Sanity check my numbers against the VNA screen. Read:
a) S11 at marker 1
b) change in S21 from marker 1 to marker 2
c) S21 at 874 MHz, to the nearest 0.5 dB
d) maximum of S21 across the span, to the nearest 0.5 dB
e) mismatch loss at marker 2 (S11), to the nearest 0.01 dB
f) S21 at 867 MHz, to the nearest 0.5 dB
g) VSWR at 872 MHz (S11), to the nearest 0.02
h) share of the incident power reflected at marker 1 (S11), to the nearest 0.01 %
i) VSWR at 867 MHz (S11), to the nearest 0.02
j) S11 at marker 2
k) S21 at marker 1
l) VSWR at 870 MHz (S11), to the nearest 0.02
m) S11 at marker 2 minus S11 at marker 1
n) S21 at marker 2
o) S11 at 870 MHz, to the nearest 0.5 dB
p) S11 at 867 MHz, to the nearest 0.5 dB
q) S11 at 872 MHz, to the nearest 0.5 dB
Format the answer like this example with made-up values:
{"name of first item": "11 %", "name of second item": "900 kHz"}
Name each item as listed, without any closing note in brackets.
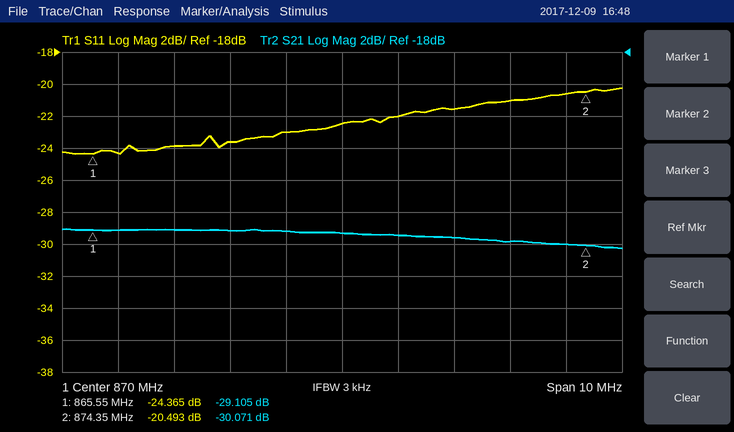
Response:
{"S11 at marker 1": "-24.365 dB", "change in S21 from marker 1 to marker 2": "-0.966 dB", "S21 at 874 MHz, to the nearest 0.5 dB": "-30.0 dB", "maximum of S21 across the span, to the nearest 0.5 dB": "-29.0 dB", "mismatch loss at marker 2 (S11), to the nearest 0.01 dB": "0.04 dB", "S21 at 867 MHz, to the nearest 0.5 dB": "-29.0 dB", "VSWR at 872 MHz (S11), to the nearest 0.02": "1.18", "share of the incident power reflected at marker 1 (S11), to the nearest 0.01 %": "0.37 %", "VSWR at 867 MHz (S11), to the nearest 0.02": "1.14", "S11 at marker 2": "-20.493 dB", "S21 at marker 1": "-29.105 dB", "VSWR at 870 MHz (S11), to the nearest 0.02": "1.16", "S11 at marker 2 minus S11 at marker 1": "3.872 dB", "S21 at marker 2": "-30.071 dB", "S11 at 870 MHz, to the nearest 0.5 dB": "-22.5 dB", "S11 at 867 MHz, to the nearest 0.5 dB": "-24.0 dB", "S11 at 872 MHz, to the nearest 0.5 dB": "-21.5 dB"}
